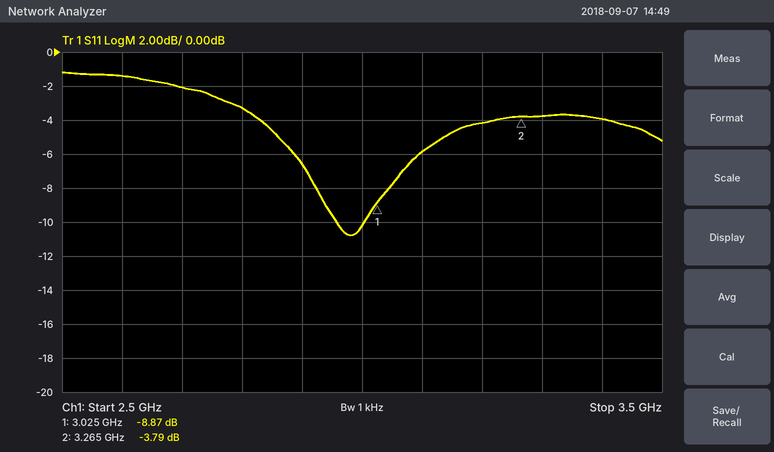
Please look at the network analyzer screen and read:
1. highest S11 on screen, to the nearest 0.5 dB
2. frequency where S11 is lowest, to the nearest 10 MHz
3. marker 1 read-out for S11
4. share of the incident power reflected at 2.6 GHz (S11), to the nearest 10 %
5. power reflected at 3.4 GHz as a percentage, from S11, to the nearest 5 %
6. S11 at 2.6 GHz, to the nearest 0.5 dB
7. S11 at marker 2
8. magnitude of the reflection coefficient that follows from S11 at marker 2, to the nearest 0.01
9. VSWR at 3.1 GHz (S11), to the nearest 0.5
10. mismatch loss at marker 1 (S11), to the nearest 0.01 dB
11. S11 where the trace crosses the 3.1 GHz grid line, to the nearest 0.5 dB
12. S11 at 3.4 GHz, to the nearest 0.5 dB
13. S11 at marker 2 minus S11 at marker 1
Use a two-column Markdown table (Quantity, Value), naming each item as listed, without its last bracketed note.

| Quantity | Value |
|---|---|
| highest S11 on screen, to the nearest 0.5 dB | -1.0 dB |
| frequency where S11 is lowest, to the nearest 10 MHz | 2.98 GHz |
| marker 1 read-out for S11 | -8.87 dB |
| share of the incident power reflected at 2.6 GHz (S11), to the nearest 10 % | 70 % |
| power reflected at 3.4 GHz as a percentage, from S11, to the nearest 5 % | 40 % |
| S11 at 2.6 GHz, to the nearest 0.5 dB | -1.5 dB |
| S11 at marker 2 | -3.79 dB |
| magnitude of the reflection coefficient that follows from S11 at marker 2, to the nearest 0.01 | 0.65 |
| VSWR at 3.1 GHz (S11), to the nearest 0.5 | 3.0 |
| mismatch loss at marker 1 (S11), to the nearest 0.01 dB | 0.60 dB |
| S11 where the trace crosses the 3.1 GHz grid line, to the nearest 0.5 dB | -6.0 dB |
| S11 at 3.4 GHz, to the nearest 0.5 dB | -4.0 dB |
| S11 at marker 2 minus S11 at marker 1 | 5.08 dB |
